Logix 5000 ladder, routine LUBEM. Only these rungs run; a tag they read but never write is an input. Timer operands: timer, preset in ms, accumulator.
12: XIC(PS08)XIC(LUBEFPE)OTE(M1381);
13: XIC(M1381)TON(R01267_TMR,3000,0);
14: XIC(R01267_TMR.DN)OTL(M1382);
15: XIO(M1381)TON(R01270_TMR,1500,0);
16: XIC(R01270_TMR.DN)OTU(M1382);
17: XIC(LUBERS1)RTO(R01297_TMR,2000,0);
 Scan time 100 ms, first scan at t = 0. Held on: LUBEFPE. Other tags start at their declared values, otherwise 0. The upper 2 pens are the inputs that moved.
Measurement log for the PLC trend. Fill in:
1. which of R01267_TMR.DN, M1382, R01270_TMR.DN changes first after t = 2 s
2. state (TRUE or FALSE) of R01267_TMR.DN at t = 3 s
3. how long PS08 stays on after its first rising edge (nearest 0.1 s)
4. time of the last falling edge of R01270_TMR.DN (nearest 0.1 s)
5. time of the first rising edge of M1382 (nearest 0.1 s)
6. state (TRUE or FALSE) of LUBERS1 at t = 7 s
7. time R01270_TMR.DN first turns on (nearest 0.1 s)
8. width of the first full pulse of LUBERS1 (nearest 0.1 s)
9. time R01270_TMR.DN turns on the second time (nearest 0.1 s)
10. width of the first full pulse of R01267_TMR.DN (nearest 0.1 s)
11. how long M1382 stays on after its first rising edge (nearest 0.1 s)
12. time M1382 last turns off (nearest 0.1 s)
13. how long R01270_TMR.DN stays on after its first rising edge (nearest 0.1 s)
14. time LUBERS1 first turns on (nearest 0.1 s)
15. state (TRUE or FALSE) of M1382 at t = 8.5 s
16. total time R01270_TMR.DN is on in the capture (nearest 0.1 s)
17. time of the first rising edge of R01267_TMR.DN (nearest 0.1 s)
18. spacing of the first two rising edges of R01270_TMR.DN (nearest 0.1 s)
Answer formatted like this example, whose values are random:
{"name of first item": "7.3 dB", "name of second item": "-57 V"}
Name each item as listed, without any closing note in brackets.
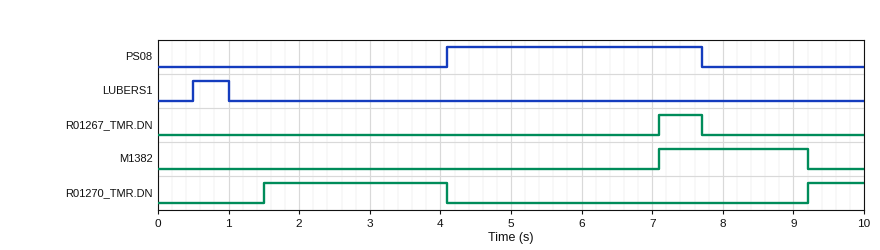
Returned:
{"which of R01267_TMR.DN, M1382, R01270_TMR.DN changes first after t = 2 s": "R01270_TMR.DN", "state (TRUE or FALSE) of R01267_TMR.DN at t = 3 s": "FALSE", "how long PS08 stays on after its first rising edge": "3.6 s", "time of the last falling edge of R01270_TMR.DN": "4.1 s", "time of the first rising edge of M1382": "7.1 s", "state (TRUE or FALSE) of LUBERS1 at t = 7 s": "FALSE", "time R01270_TMR.DN first turns on": "1.5 s", "width of the first full pulse of LUBERS1": "0.5 s", "time R01270_TMR.DN turns on the second time": "9.2 s", "width of the first full pulse of R01267_TMR.DN": "0.6 s", "how long M1382 stays on after its first rising edge": "2.1 s", "time M1382 last turns off": "9.2 s", "how long R01270_TMR.DN stays on after its first rising edge": "2.6 s", "time LUBERS1 first turns on": "0.5 s", "state (TRUE or FALSE) of M1382 at t = 8.5 s": "TRUE", "total time R01270_TMR.DN is on in the capture": "3.4 s", "time of the first rising edge of R01267_TMR.DN": "7.1 s", "spacing of the first two rising edges of R01270_TMR.DN": "7.7 s"}
